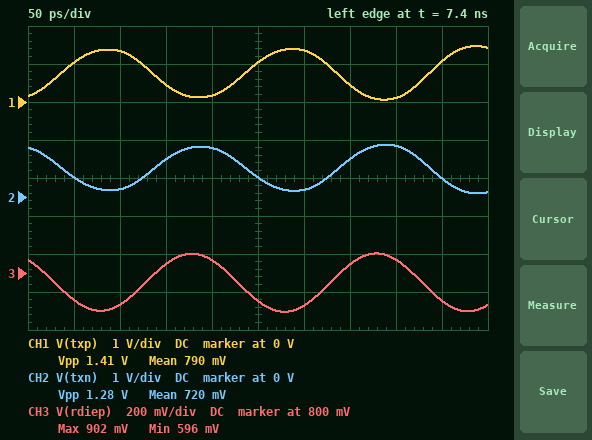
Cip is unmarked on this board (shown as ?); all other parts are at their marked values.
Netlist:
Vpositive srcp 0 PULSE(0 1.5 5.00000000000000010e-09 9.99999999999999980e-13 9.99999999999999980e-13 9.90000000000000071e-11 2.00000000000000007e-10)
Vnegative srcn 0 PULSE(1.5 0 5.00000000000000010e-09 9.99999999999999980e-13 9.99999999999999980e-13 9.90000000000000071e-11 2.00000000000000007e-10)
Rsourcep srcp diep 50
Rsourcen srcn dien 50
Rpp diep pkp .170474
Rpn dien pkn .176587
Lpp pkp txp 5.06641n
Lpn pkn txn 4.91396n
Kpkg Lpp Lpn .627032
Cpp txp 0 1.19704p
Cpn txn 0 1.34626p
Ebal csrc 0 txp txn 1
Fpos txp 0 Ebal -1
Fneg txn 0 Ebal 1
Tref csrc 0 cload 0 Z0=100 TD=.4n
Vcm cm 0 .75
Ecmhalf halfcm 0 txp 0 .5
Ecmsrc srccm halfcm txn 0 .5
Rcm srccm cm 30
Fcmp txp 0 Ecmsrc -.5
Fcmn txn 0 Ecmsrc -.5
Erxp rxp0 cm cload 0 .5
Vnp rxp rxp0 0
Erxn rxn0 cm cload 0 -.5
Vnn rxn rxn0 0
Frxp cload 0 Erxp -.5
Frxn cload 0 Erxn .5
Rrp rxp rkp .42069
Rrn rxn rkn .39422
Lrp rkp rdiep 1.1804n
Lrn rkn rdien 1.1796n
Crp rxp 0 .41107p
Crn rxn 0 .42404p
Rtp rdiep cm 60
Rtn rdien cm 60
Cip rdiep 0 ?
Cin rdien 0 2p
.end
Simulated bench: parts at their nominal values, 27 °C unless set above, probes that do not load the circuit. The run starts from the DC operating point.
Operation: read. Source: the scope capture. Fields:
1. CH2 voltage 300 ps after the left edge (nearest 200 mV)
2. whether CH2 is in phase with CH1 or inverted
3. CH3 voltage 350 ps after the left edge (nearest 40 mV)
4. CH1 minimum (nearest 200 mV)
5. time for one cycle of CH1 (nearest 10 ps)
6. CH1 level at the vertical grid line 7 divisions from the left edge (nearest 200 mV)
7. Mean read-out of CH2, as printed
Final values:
200 mV
inverted
840 mV
0 V
200 ps
400 mV
720 mV
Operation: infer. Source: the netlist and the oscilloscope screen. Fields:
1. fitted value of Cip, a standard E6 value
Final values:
4.7 pF
